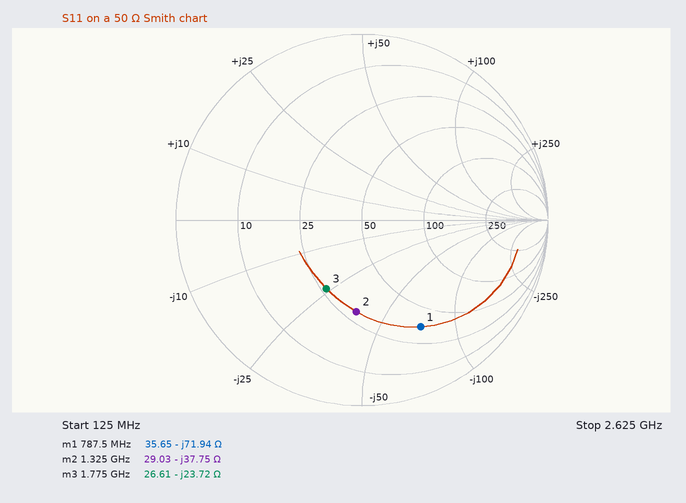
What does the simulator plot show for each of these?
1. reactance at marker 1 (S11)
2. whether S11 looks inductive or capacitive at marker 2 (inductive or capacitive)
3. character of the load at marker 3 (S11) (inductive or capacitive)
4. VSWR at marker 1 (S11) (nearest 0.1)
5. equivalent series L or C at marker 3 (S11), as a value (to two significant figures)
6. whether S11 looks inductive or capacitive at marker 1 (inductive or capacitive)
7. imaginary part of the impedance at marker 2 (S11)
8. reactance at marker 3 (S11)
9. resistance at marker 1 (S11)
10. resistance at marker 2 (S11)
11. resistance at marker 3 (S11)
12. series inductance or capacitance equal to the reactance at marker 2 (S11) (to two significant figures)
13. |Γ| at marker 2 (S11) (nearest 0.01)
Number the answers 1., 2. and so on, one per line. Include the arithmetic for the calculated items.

1. -71.94 Ω
2. capacitive
3. capacitive
4. 4.8
5. C = 1/(2π × 1.775 GHz × 23.72 Ω) ≈ 3.8 pF
6. capacitive
7. -37.75 Ω
8. -23.72 Ω
9. 35.65 Ω
10. 29.03 Ω
11. 26.61 Ω
12. C = 1/(2π × 1.325 GHz × 37.75 Ω) ≈ 3.2 pF
13. 0.49
